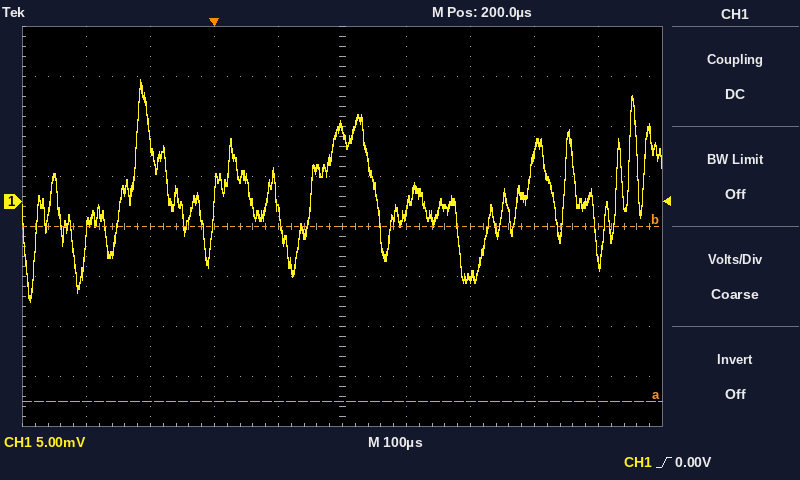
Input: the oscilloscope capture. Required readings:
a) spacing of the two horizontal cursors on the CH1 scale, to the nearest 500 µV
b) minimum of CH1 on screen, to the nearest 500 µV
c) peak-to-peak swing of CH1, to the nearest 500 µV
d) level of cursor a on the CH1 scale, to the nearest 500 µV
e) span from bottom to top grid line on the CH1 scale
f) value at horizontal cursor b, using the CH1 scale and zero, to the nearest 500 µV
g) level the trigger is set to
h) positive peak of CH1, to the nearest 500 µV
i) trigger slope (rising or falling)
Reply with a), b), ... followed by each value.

a) 17.5 mV
b) -10.0 mV
c) 22.0 mV
d) -20.0 mV
e) 40 mV
f) -2.5 mV
g) 0.00 V
h) 12.0 mV
i) rising
